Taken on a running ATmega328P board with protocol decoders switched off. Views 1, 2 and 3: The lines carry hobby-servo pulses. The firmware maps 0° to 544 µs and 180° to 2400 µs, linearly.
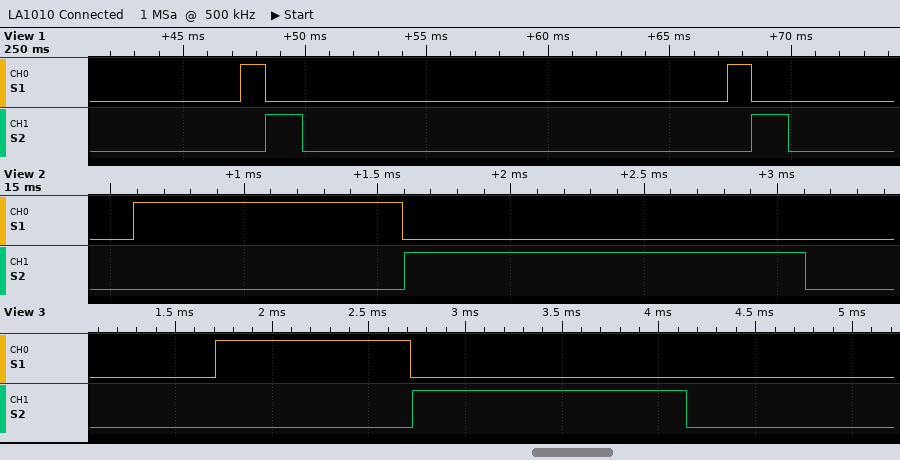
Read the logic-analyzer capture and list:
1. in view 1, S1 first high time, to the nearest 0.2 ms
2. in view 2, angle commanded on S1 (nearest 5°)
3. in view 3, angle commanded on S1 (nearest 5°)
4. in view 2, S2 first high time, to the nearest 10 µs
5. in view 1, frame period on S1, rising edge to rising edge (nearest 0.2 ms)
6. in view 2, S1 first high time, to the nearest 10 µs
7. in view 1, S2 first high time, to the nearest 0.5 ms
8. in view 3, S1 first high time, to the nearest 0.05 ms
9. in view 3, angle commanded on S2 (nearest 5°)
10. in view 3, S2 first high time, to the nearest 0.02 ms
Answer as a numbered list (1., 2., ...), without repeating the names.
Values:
1. 1.0 ms
2. 45°
3. 45°
4. 1500 µs
5. 20.0 ms
6. 1010 µs
7. 1.5 ms
8. 1.00 ms
9. 85°
10. 1.42 ms
